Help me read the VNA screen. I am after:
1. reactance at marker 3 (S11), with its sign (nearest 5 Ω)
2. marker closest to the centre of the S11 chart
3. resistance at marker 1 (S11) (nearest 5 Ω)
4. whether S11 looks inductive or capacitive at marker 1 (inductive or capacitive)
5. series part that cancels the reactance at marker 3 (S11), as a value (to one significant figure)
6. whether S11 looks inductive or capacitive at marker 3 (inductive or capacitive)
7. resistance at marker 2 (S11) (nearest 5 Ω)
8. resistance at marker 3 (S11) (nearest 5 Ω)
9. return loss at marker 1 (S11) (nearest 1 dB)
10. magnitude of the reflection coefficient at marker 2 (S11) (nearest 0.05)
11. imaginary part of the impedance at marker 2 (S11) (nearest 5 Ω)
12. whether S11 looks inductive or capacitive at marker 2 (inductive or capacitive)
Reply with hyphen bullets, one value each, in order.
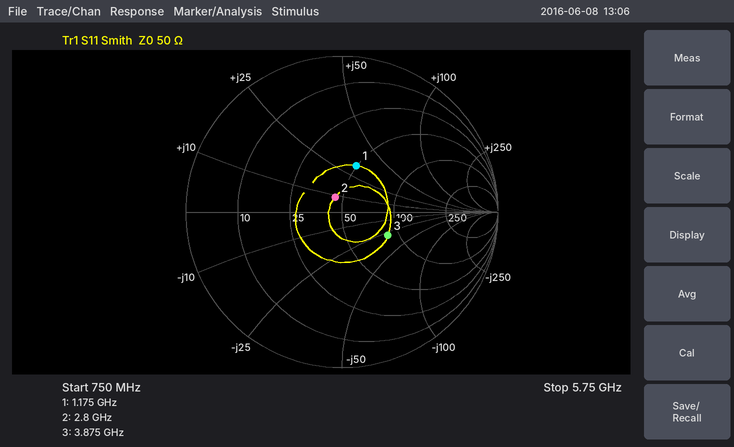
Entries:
- -30 Ω
- marker 2
- 50 Ω
- inductive
- 1 nH
- capacitive
- 45 Ω
- 85 Ω
- 10 dB
- 0.10
- +10 Ω
- inductive
